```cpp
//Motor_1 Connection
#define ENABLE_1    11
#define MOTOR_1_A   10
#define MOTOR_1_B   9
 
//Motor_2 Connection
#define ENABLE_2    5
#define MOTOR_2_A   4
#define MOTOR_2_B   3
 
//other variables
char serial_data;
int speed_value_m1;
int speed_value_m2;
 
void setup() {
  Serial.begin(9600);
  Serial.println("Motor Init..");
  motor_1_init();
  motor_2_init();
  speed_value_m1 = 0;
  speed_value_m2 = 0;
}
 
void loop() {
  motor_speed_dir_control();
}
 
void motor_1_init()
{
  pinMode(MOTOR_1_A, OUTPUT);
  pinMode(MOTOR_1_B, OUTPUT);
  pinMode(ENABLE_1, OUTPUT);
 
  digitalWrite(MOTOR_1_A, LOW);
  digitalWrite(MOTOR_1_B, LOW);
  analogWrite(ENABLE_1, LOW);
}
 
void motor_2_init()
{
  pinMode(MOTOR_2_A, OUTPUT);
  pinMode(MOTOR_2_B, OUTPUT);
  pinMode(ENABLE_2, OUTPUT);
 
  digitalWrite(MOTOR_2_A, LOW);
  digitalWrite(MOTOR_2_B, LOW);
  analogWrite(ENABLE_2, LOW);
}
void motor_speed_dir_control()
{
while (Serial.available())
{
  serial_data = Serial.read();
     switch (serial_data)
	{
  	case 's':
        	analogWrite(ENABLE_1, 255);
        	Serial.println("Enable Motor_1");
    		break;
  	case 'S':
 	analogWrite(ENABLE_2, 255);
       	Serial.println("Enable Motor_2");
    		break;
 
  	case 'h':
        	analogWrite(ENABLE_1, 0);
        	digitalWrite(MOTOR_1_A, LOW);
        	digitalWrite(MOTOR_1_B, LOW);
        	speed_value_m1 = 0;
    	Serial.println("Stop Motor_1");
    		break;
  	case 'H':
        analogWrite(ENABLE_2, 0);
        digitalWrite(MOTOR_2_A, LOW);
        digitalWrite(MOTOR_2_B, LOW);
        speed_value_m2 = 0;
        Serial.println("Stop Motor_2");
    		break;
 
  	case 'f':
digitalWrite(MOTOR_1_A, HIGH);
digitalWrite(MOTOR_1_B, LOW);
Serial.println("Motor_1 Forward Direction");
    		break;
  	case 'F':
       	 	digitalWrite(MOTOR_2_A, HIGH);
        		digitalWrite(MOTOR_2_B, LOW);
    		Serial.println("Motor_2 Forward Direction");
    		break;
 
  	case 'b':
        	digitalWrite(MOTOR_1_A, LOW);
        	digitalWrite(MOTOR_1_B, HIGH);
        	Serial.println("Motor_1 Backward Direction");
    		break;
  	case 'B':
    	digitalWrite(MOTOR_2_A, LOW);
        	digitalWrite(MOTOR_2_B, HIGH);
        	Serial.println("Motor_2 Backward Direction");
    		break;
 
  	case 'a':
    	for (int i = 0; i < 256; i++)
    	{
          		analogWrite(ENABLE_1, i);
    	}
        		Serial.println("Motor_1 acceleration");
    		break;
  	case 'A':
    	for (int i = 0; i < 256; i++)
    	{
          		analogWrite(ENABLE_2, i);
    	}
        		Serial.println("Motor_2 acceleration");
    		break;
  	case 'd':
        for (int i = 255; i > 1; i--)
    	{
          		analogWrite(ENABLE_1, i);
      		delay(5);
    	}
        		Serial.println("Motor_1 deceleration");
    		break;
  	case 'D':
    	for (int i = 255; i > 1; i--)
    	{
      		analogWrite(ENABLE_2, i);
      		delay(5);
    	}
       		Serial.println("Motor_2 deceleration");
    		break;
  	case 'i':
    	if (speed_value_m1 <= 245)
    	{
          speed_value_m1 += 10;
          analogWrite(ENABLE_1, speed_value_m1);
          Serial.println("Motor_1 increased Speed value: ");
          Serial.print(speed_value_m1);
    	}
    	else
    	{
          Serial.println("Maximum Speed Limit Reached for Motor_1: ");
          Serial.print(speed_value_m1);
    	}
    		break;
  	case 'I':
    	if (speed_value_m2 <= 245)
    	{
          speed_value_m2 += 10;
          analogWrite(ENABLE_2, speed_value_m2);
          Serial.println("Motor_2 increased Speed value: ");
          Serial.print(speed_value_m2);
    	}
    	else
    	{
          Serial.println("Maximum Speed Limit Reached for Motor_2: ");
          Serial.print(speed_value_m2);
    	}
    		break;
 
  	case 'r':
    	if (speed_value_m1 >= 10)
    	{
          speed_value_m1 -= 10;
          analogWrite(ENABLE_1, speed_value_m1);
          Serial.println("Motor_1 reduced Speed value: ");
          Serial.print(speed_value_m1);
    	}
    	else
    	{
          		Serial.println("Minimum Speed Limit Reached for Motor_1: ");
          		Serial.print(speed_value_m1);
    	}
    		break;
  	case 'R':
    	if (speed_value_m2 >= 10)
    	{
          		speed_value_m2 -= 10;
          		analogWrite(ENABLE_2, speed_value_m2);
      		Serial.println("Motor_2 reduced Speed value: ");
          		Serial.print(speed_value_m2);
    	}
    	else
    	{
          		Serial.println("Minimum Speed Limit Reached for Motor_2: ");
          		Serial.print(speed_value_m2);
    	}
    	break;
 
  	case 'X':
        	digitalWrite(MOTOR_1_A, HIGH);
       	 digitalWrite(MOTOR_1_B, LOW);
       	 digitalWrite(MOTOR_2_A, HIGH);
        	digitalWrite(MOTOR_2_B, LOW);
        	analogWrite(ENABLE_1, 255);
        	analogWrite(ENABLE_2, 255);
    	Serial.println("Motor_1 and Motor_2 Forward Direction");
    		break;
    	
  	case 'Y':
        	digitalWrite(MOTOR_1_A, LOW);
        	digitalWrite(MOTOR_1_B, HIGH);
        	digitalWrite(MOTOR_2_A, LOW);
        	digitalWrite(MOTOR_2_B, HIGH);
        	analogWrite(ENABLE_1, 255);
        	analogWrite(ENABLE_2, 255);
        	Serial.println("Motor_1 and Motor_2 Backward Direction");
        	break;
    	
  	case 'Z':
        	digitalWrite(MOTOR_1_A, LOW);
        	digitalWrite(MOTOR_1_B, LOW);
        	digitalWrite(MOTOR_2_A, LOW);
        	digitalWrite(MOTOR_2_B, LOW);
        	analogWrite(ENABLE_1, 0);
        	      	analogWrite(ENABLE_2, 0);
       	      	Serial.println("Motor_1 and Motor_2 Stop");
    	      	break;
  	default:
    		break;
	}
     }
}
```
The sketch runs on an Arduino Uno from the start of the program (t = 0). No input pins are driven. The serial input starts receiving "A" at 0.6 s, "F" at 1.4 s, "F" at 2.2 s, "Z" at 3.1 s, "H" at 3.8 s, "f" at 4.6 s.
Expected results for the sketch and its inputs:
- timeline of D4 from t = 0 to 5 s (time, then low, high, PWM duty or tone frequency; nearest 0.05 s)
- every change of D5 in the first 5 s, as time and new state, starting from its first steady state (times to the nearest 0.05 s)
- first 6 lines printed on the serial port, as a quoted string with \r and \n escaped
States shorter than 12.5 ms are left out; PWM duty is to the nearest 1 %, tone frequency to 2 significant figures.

0 s low; 1.4 s high; 3.1 s low
0 s low; 0.6 s high; 3.1 s low
"Motor Init..\r\nMotor_2 acceleration\r\nMotor_2 Forward Direction\r\nMotor_2 Forward Direction\r\nMotor_1 and Motor_2 Stop\r\nStop Motor_2\r\n"
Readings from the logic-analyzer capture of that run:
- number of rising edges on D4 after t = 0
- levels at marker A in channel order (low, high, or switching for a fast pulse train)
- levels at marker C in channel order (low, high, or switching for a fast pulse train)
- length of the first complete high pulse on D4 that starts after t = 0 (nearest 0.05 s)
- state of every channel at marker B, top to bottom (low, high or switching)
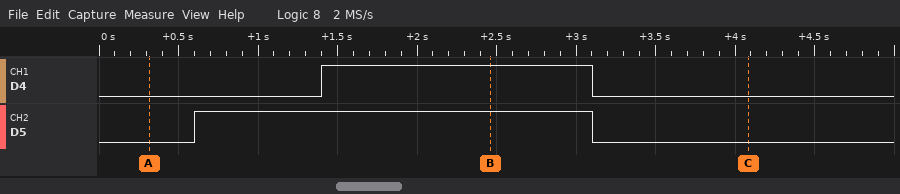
1
D4 low, D5 low
D4 low, D5 low
1.70 s
D4 high, D5 high
